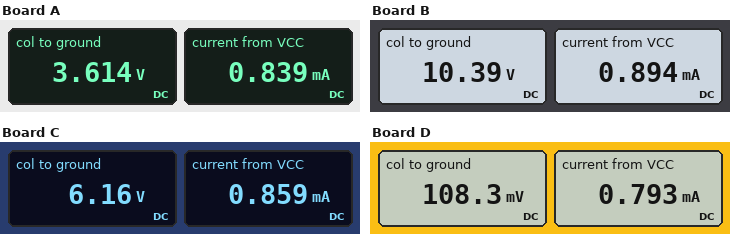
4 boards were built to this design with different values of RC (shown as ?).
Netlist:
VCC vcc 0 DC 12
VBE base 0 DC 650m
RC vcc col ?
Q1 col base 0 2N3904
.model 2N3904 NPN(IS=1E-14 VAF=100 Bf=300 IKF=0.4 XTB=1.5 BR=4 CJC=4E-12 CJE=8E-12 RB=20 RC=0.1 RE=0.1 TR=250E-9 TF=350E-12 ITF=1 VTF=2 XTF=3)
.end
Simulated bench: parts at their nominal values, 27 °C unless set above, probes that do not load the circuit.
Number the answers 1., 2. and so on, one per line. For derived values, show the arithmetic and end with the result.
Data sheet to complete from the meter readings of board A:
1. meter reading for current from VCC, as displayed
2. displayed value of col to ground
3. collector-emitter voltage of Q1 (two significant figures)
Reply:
1. 0.839 mA
2. 3.614 V
3. 3.614 V = 3.6 V
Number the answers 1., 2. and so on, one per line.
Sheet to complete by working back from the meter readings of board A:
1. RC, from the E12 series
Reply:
1. 10 kΩ
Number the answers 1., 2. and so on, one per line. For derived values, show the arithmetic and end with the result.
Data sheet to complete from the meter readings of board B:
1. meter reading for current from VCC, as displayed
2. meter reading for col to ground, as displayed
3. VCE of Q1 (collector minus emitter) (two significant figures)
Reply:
1. 0.894 mA
2. 10.39 V
3. 10.39 V = 10 V
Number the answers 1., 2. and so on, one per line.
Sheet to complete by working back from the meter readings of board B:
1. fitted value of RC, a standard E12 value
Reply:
1. 1.8 kΩ
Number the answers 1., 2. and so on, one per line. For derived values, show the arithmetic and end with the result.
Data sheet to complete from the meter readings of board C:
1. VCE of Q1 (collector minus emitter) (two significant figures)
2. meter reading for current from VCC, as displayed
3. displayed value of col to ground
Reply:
1. 6.16 V = 6.2 V
2. 0.859 mA
3. 6.16 V
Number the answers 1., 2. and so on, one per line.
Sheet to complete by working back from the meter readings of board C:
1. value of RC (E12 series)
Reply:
1. 6.8 kΩ
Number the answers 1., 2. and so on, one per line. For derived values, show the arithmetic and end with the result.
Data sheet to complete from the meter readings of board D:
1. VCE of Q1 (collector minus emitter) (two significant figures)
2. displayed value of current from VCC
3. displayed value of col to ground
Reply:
1. 108.3 mV = 110 mV
2. 0.793 mA
3. 108.3 mV
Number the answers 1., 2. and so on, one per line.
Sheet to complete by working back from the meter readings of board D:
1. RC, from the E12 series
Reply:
1. 15 kΩ
